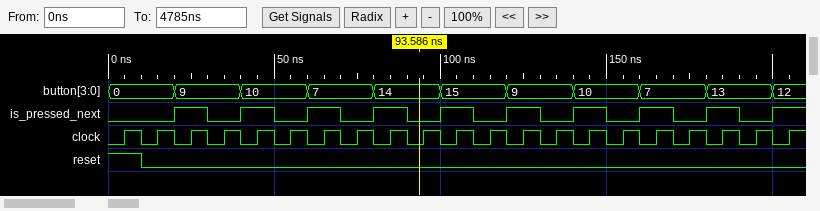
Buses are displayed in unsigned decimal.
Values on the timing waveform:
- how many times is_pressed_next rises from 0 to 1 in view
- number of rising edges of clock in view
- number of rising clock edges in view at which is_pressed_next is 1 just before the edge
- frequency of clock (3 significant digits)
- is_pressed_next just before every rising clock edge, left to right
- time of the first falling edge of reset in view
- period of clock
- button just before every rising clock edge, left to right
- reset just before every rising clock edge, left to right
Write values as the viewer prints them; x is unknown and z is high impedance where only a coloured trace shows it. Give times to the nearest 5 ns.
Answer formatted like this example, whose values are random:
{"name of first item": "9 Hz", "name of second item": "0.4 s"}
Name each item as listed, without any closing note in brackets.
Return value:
{"how many times is_pressed_next rises from 0 to 1 in view": "10", "number of rising edges of clock in view": "21", "number of rising clock edges in view at which is_pressed_next is 1 just before the edge": "10", "frequency of clock": "100 MHz", "is_pressed_next just before every rising clock edge, left to right": "0 0 1 0 1 0 1 0 1 0 1 0 1 0 1 0 1 0 1 0 1", "time of the first falling edge of reset in view": "10 ns", "period of clock": "10 ns", "button just before every rising clock edge, left to right": "0, 0, 9, 9, 10, 10, 7, 7, 14, 14, 15, 15, 9, 9, 10, 10, 7, 7, 13, 13, 12", "reset just before every rising clock edge, left to right": "1 0 0 0 0 0 0 0 0 0 0 0 0 0 0 0 0 0 0 0 0"}
